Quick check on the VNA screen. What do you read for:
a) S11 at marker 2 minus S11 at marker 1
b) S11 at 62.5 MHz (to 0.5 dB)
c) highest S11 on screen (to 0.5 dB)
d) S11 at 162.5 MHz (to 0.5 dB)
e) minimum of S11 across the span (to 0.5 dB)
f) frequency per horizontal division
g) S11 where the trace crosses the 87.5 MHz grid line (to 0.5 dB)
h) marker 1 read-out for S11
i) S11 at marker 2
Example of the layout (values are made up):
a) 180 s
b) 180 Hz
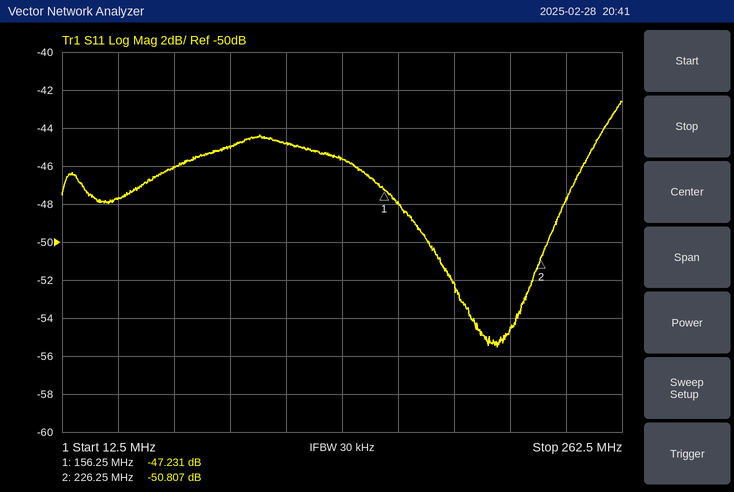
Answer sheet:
a) -3.576 dB
b) -46.0 dB
c) -42.5 dB
d) -48.0 dB
e) -55.5 dB
f) 25 MHz
g) -45.0 dB
h) -47.231 dB
i) -50.807 dB
